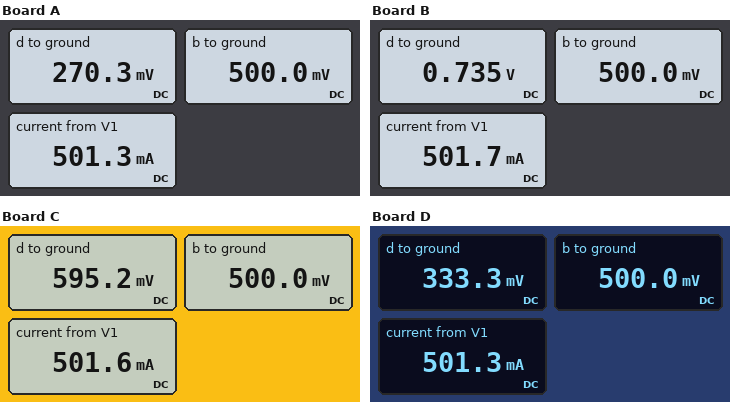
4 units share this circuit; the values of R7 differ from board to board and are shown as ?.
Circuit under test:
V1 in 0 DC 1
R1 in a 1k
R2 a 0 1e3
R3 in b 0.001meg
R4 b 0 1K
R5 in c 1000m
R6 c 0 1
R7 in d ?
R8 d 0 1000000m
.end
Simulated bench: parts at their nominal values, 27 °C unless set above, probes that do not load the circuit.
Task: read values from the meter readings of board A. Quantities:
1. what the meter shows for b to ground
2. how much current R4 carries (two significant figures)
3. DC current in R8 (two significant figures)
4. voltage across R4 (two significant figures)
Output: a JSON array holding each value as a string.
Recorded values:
["500.0 mV", "500 µA", "270 µA", "500 mV"]
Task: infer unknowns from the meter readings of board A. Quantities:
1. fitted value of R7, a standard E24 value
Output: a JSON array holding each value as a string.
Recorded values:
["2.7 kΩ"]
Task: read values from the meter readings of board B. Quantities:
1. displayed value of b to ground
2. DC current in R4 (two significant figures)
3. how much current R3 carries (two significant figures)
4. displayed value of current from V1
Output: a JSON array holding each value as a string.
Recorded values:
["500.0 mV", "500 µA", "500 µA", "501.7 mA"]
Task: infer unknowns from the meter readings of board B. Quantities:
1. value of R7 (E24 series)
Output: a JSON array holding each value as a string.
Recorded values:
["360 Ω"]
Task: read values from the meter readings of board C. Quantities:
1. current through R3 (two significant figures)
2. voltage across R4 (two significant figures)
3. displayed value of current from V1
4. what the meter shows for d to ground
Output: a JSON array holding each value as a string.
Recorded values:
["500 µA", "500 mV", "501.6 mA", "595.2 mV"]
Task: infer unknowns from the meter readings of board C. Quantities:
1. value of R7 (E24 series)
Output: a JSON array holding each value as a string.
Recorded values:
["680 Ω"]
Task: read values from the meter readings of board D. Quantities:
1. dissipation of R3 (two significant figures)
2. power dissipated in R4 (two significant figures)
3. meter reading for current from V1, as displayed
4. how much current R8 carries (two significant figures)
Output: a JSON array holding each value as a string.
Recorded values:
["250 µW", "250 µW", "501.3 mA", "330 µA"]
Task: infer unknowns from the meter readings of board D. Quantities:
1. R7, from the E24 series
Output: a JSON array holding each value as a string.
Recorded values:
["2 kΩ"]
